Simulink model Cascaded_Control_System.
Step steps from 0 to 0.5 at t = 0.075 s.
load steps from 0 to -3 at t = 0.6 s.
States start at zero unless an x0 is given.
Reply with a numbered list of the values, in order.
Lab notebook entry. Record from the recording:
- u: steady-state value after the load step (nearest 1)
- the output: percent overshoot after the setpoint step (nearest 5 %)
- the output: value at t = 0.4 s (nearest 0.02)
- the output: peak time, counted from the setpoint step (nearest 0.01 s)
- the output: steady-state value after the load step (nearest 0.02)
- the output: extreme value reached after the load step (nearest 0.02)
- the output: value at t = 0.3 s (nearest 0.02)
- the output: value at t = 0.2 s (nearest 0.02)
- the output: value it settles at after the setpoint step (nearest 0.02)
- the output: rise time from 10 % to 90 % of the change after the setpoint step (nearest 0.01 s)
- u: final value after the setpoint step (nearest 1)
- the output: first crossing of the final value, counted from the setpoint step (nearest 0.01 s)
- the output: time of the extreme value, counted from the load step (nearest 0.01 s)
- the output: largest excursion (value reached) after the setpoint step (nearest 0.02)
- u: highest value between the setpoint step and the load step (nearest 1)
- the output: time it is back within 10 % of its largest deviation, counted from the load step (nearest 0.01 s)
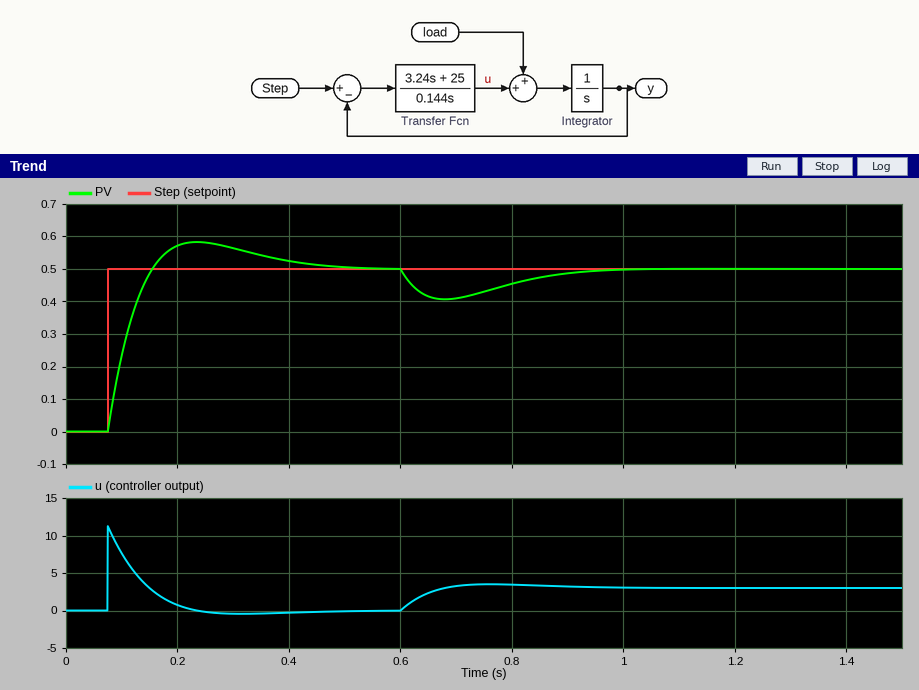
1. 3
2. 15 %
3. 0.52
4. 0.16 s
5. 0.50
6. 0.40
7. 0.56
8. 0.58
9. 0.50
10. 0.06 s
11. 0
12. 0.08 s
13. 0.08 s
14. 0.58
15. 11
16. 0.32 s
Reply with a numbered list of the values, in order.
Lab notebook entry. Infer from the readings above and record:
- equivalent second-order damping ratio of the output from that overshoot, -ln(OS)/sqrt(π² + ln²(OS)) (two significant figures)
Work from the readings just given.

1. 0.52
